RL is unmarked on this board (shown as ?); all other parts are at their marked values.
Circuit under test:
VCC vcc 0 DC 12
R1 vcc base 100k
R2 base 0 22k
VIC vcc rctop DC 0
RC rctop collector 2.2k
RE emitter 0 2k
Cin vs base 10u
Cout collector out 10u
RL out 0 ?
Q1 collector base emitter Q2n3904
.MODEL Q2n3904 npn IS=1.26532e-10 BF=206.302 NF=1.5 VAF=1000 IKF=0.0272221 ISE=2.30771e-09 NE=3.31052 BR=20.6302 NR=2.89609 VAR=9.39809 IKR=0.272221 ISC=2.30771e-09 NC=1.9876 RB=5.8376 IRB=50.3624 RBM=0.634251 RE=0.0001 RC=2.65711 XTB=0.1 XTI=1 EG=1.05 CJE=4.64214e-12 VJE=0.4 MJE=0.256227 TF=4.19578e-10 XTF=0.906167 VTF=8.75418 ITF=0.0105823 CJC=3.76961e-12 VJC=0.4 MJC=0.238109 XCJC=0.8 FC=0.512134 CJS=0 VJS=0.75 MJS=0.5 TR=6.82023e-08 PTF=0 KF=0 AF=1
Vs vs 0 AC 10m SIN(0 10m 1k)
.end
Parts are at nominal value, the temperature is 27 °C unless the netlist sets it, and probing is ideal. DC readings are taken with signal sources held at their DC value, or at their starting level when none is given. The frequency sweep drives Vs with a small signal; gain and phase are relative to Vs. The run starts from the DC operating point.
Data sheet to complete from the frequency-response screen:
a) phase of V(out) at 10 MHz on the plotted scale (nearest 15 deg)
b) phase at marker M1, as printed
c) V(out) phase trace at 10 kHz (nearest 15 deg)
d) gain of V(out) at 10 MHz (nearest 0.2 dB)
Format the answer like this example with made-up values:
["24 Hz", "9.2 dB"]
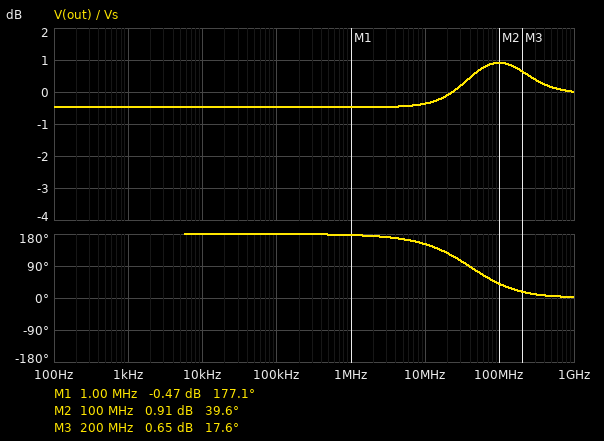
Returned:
["150 deg", "177.1 deg", "180 deg", "-0.4 dB"]
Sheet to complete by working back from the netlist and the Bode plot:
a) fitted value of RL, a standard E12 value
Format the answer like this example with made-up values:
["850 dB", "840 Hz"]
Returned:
["18 kΩ"]
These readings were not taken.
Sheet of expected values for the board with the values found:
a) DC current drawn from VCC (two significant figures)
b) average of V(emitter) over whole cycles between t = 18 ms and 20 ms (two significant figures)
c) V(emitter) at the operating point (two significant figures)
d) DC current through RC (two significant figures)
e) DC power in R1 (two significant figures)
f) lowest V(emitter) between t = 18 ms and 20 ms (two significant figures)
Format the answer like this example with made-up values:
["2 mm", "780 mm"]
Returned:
["810 µA", "1.4 V", "1.4 V", "710 µA", "990 µW", "1.4 V"]
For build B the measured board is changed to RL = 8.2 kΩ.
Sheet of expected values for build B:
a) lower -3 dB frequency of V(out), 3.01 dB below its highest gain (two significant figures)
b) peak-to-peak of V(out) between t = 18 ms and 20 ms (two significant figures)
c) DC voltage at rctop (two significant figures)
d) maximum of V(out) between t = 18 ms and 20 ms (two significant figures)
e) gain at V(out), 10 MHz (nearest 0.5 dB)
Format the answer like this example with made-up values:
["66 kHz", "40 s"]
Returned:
["4.3 Hz", "17 mV", "12 V", "8.4 mV", "-1.5 dB"]
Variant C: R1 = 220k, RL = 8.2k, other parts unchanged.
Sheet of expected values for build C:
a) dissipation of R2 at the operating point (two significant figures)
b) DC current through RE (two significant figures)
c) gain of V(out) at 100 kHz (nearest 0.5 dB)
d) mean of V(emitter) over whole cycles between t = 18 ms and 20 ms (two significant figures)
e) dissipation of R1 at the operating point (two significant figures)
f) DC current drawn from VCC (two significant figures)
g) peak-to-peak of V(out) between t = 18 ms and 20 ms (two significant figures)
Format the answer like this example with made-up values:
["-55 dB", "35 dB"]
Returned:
["49 µW", "240 µA", "-2.0 dB", "470 mV", "550 µW", "280 µA", "16 mV"]
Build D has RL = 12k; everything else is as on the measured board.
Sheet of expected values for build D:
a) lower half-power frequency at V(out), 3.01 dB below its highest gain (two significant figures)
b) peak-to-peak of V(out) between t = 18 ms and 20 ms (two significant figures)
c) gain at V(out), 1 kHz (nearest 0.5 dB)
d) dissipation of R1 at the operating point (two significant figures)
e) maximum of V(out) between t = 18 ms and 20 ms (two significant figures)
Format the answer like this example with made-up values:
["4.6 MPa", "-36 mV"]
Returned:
["2.6 Hz", "18 mV", "-1.0 dB", "990 µW", "9.0 mV"]
